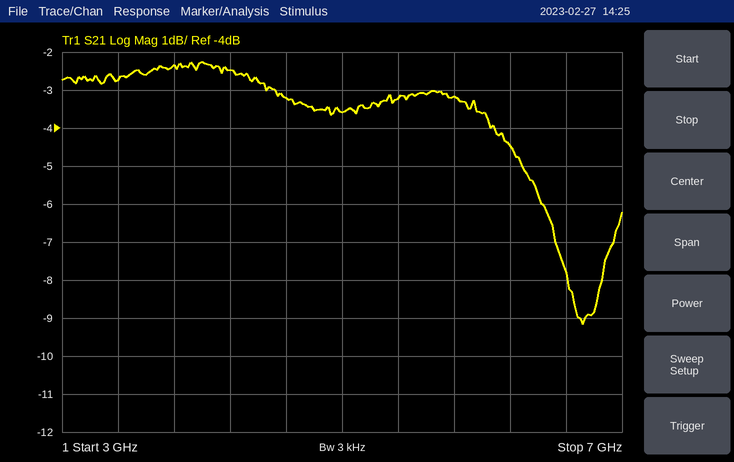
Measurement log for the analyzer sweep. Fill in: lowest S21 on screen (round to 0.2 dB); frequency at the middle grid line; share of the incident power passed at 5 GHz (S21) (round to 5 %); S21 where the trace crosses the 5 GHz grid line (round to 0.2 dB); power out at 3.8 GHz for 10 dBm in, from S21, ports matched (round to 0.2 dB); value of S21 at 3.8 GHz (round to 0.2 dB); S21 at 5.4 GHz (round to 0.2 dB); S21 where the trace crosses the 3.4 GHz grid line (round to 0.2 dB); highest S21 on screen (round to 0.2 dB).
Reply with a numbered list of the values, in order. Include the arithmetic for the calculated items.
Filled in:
1. -9.2 dB
2. 5 GHz
3. 10^(-3.6/10) ≈ 43.7 %, so 45 % to the nearest 5 %
4. -3.6 dB
5. 10 dBm + (-2.4 dB) = 7.6 dBm
6. -2.4 dB
7. -3.2 dB
8. -2.8 dB
9. -2.2 dB
